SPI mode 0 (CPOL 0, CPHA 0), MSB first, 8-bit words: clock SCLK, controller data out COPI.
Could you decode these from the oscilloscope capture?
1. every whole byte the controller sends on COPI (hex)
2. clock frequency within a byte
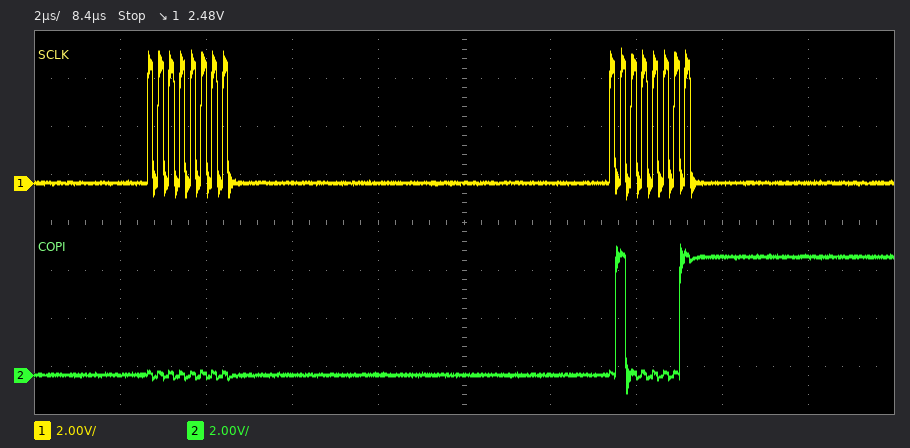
00 41
4 MHz
